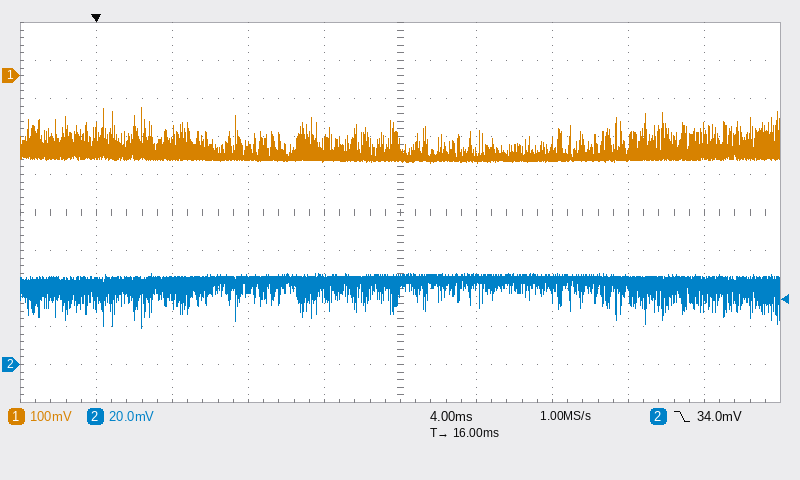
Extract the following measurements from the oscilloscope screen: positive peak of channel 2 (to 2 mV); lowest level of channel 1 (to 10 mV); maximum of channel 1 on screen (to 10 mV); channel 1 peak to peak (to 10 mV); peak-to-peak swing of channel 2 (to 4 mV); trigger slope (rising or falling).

48 mV
-230 mV
-80 mV
150 mV
28 mV
falling
